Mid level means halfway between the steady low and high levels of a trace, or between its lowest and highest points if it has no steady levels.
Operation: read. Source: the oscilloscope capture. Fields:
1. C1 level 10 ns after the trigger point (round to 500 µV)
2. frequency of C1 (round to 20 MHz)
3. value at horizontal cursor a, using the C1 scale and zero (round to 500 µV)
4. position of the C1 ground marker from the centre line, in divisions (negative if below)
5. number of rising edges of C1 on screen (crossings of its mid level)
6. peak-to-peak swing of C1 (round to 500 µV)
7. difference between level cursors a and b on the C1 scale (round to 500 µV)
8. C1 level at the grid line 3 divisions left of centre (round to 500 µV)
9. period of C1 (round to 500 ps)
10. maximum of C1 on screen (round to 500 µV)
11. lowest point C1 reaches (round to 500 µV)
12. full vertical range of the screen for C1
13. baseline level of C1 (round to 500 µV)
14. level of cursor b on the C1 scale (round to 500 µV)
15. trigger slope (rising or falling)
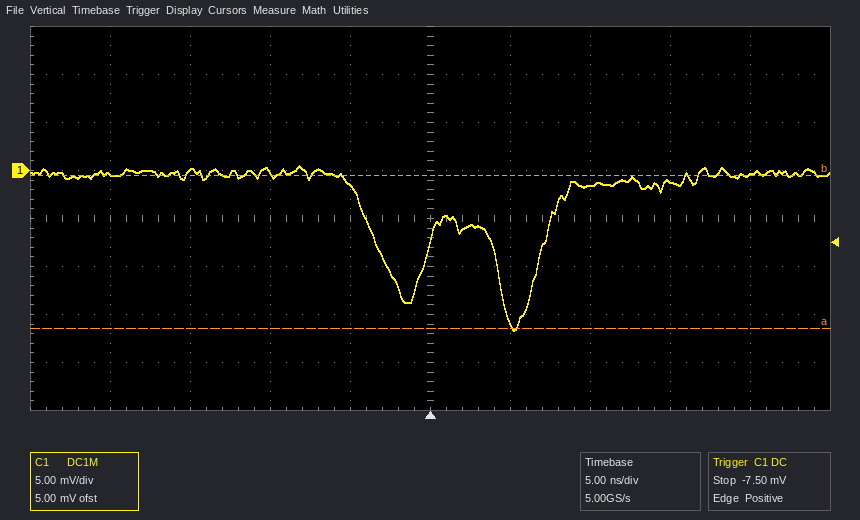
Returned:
-1.5 mV
140 MHz
-16.5 mV
+1.0 div
2
17.0 mV
16.0 mV
0.0 mV
7.0 ns
500 µV
-16.5 mV
40 mV
-500 µV
-500 µV
rising
